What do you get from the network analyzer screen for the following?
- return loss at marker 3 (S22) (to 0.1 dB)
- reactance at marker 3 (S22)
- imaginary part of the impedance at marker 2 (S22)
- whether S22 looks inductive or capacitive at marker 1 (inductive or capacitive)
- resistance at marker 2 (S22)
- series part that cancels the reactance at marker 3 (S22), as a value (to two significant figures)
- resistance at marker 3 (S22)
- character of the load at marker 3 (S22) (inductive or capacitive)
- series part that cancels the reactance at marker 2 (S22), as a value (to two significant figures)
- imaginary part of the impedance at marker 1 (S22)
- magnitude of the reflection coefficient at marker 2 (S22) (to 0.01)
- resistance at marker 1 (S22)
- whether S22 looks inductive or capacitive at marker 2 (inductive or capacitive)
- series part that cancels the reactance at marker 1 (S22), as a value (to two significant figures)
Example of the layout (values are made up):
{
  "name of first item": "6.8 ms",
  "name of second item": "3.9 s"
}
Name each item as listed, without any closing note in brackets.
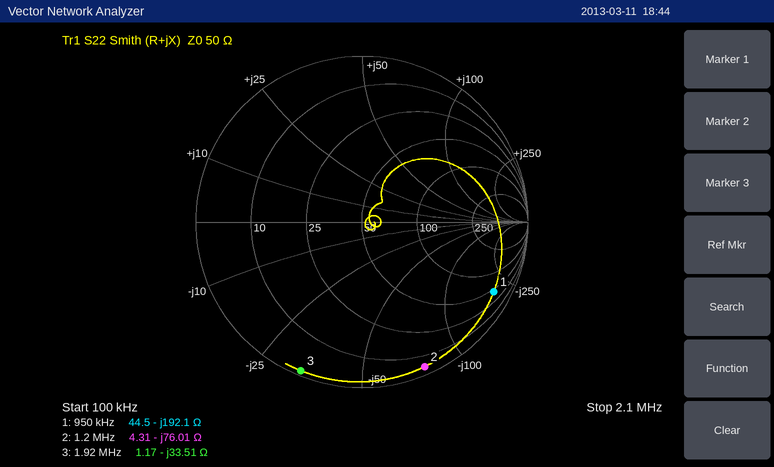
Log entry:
{
  "return loss at marker 3 (S22)": "0.3 dB",
  "reactance at marker 3": "-33.51 Ω",
  "imaginary part of the impedance at marker 2": "-76.01 Ω",
  "whether S22 looks inductive or capacitive at marker 1": "capacitive",
  "resistance at marker 2": "4.31 Ω",
  "series part that cancels the reactance at marker 3 (S22), as a value": "2.8 µH",
  "resistance at marker 3": "1.17 Ω",
  "character of the load at marker 3 (S22)": "capacitive",
  "series part that cancels the reactance at marker 2 (S22), as a value": "10 µH",
  "imaginary part of the impedance at marker 1": "-192.1 Ω",
  "magnitude of the reflection coefficient at marker 2 (S22)": "0.95",
  "resistance at marker 1": "44.5 Ω",
  "whether S22 looks inductive or capacitive at marker 2": "capacitive",
  "series part that cancels the reactance at marker 1 (S22), as a value": "32 µH"
}
